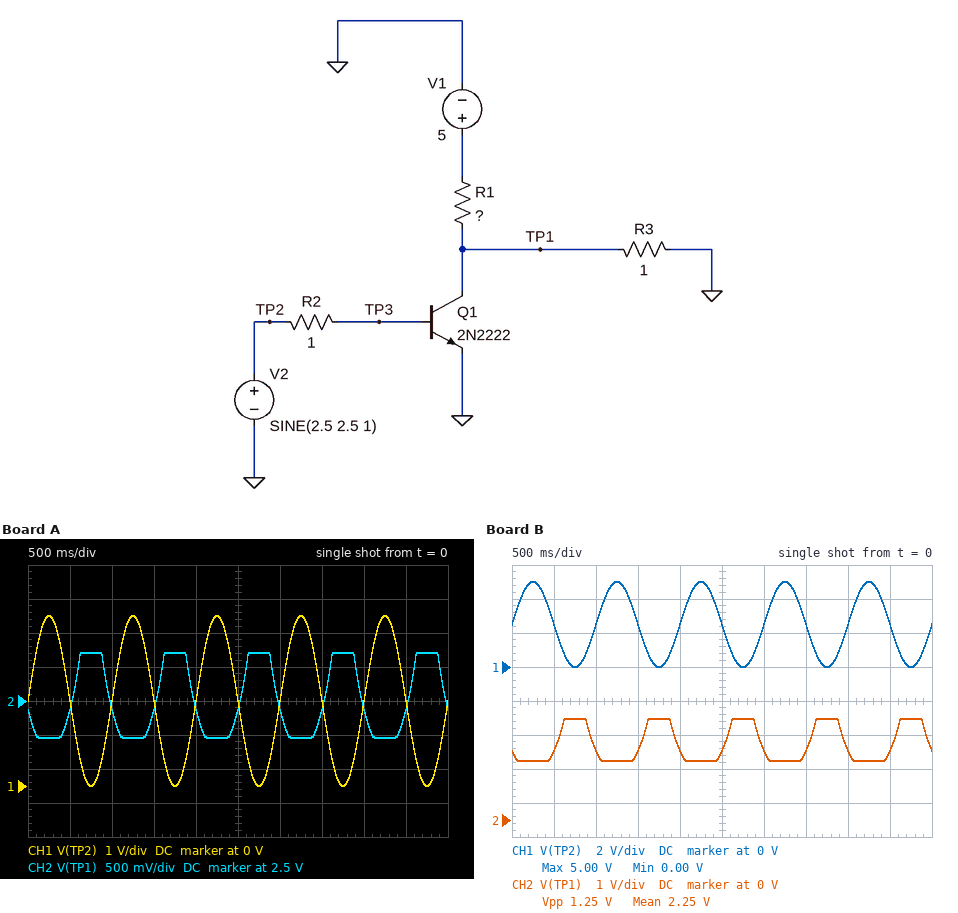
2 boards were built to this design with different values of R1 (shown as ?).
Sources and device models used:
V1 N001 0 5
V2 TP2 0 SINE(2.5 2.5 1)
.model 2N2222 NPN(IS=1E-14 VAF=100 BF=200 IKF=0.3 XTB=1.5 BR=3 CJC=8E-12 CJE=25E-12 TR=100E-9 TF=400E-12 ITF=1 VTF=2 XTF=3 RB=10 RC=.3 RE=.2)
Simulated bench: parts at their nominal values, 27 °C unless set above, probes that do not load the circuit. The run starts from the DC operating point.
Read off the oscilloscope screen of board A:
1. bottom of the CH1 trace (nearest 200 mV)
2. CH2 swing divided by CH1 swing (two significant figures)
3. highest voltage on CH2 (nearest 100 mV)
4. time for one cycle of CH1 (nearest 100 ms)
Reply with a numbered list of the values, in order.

1. 0 V
2. 0.25
3. 3.2 V
4. 1.0 s
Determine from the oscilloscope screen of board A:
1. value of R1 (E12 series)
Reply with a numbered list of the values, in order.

1. 0.56 Ω
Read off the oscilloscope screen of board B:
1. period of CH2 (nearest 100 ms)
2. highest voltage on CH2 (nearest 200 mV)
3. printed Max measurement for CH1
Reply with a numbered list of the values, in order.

1. 1.0 s
2. 3.0 V
3. 5.00 V
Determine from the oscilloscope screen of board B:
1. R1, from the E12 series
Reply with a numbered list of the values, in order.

1. 0.68 Ω
